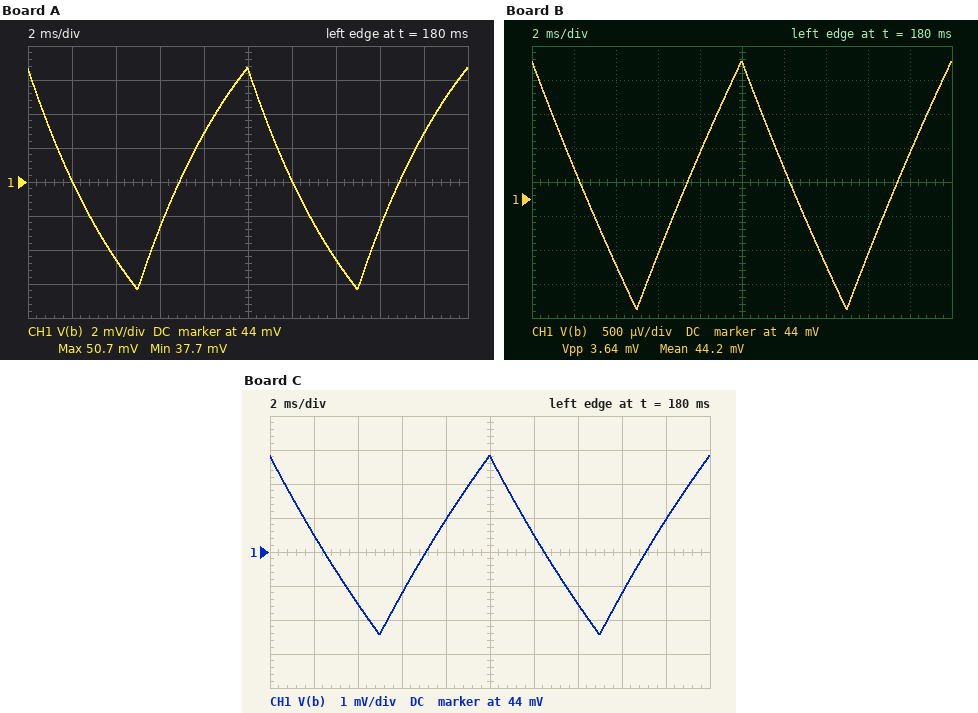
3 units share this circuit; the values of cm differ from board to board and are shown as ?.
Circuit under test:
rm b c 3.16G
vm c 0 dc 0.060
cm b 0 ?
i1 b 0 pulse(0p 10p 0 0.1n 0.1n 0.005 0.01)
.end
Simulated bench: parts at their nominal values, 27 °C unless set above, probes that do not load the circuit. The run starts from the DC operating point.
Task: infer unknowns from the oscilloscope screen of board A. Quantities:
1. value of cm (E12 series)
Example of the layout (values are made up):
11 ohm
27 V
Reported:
1.8 pF
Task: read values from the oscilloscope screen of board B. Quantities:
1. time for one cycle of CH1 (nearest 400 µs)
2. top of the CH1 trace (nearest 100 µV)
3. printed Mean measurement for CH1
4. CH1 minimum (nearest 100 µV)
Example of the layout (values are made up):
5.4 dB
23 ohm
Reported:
10.0 ms
46.0 mV
44.2 mV
42.4 mV
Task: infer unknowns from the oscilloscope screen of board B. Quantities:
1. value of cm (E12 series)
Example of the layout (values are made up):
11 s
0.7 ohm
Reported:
6.8 pF
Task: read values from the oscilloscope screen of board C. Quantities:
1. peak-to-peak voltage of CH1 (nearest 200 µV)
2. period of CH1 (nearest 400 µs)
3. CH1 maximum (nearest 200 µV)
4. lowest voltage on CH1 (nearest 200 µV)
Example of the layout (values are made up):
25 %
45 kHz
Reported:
5.2 mV
10.0 ms
46.8 mV
41.6 mV
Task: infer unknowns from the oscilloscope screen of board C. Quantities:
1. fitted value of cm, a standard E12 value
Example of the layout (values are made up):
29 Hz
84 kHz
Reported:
4.7 pF
